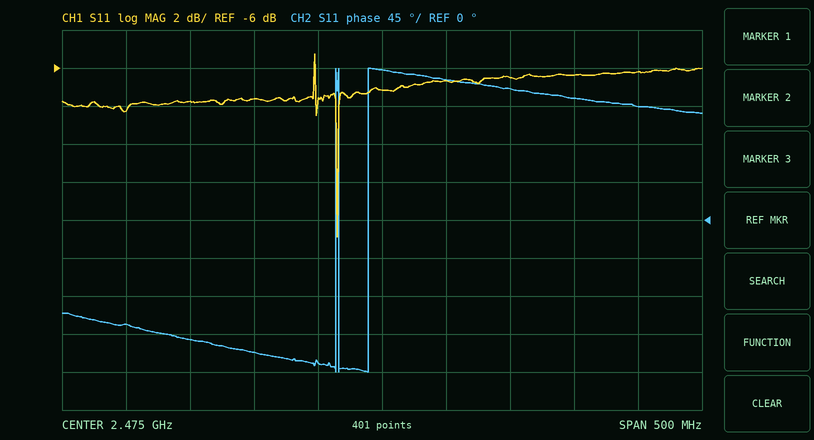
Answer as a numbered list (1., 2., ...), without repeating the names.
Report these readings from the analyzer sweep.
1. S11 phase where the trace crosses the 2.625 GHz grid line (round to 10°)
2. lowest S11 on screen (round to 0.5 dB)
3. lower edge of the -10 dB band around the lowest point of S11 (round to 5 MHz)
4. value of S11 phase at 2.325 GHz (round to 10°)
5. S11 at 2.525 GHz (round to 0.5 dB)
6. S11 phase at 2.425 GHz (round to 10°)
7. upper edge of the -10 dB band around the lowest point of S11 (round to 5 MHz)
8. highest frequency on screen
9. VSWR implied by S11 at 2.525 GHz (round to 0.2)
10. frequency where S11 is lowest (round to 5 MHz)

1. 140°
2. -15.0 dB
3. 2.440 GHz
4. -140°
5. -6.5 dB
6. -170°
7. 2.440 GHz
8. 2.725 GHz
9. 2.8
10. 2.440 GHz
